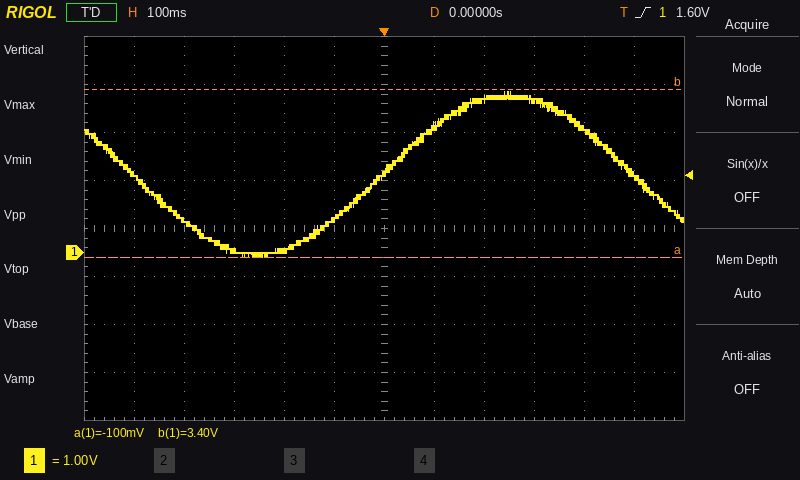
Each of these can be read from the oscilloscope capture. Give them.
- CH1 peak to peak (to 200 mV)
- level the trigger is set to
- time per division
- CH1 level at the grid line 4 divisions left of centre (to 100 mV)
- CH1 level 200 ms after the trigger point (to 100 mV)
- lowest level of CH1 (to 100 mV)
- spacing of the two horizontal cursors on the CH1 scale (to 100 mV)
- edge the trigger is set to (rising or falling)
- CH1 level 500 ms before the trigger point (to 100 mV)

3.4 V
1.60 V
100 ms
600 mV
3.2 V
-100 mV
3.5 V
rising
1.6 V
